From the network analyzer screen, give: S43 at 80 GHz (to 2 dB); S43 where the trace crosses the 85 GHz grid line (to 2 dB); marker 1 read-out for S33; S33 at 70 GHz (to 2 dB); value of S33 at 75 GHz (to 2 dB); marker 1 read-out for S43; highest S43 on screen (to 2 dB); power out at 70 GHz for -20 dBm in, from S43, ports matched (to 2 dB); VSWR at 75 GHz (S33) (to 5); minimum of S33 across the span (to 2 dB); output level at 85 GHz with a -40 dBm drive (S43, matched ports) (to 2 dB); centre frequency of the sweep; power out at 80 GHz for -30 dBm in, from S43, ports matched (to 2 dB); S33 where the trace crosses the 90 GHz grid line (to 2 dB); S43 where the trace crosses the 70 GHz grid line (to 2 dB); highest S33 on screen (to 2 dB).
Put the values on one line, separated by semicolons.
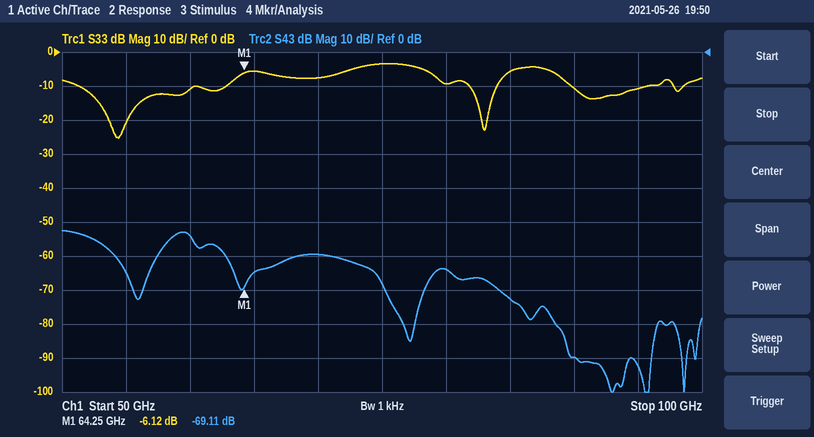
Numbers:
-64 dB; -72 dB; -6.12 dB; -8 dB; -4 dB; -69.11 dB; -52 dB; -80 dBm; 5; -26 dB; -112 dBm; 75 GHz; -94 dBm; -10 dB; -60 dB; -4 dB
